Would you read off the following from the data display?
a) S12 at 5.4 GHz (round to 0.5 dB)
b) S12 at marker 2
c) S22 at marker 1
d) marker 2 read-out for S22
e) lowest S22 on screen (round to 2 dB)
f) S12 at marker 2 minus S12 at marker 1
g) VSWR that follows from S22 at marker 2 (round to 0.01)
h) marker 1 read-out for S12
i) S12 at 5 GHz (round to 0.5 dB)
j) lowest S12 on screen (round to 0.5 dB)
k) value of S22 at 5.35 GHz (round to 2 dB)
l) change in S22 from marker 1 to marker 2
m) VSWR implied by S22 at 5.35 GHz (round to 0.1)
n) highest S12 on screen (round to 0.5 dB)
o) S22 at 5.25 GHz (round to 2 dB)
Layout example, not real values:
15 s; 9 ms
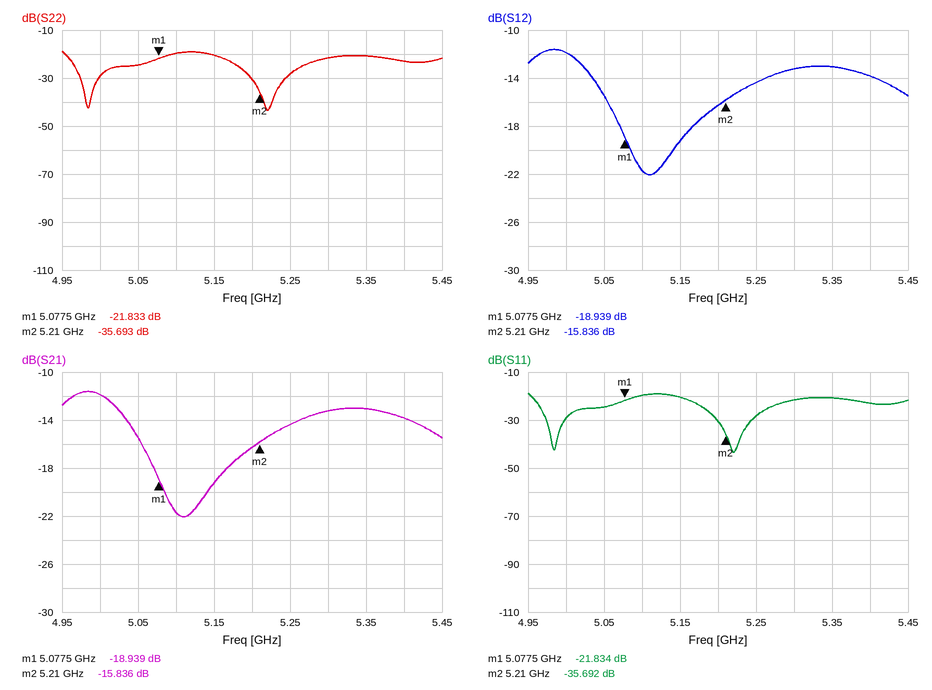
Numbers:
-14.0 dB; -15.836 dB; -21.833 dB; -35.693 dB; -44 dB; 3.103 dB; 1.03; -18.939 dB; -12.0 dB; -22.0 dB; -20 dB; -13.860 dB; 1.2; -11.5 dB; -28 dB
